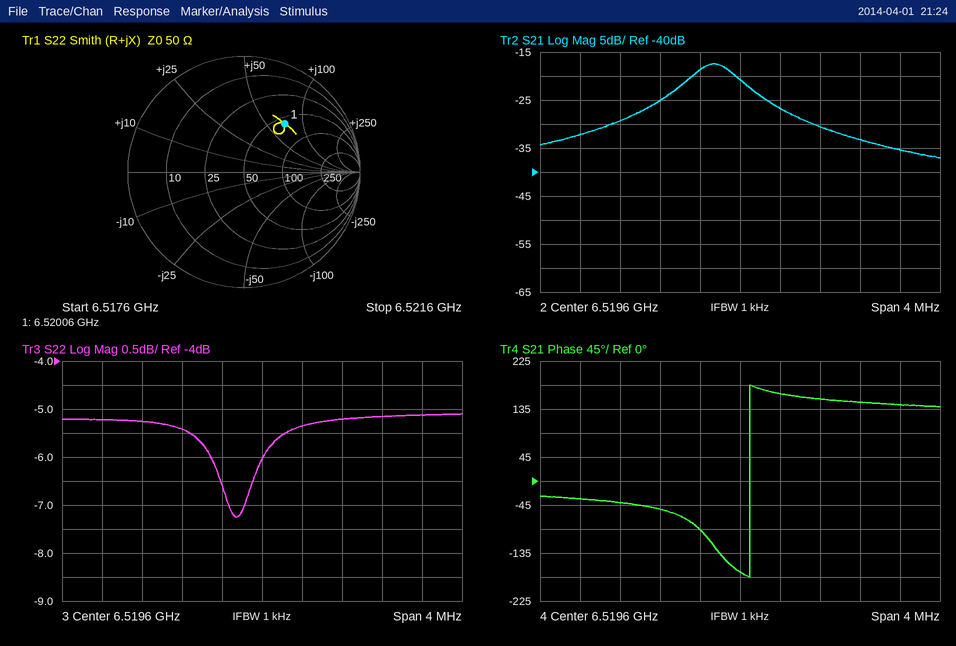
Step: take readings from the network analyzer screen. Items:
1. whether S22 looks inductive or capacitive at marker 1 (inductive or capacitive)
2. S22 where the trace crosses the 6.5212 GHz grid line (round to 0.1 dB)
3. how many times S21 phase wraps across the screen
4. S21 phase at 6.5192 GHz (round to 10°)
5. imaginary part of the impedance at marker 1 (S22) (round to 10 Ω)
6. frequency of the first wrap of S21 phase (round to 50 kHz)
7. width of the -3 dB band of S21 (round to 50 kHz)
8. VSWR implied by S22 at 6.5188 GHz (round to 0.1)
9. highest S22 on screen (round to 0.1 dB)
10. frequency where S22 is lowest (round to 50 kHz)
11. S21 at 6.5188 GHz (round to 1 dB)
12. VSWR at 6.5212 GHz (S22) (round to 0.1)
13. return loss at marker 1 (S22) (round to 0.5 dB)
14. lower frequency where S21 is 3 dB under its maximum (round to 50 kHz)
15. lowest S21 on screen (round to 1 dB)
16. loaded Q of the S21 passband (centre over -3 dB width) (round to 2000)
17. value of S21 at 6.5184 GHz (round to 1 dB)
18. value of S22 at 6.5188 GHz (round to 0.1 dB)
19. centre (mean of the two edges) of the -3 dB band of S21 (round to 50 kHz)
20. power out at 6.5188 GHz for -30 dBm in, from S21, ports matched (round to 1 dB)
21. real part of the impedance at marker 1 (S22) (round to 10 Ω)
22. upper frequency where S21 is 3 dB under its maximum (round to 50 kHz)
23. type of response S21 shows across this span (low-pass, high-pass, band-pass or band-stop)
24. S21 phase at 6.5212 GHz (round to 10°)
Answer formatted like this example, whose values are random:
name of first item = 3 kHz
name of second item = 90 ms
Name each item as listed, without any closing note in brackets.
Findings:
whether S22 looks inductive or capacitive at marker 1 = inductive
S22 where the trace crosses the 6.5212 GHz grid line = -5.1 dB
how many times S21 phase wraps across the screen = 1
S21 phase at 6.5192 GHz = -90°
imaginary part of the impedance at marker 1 (S22) = +70 Ω
frequency of the first wrap of S21 phase = 6.51970 GHz
width of the -3 dB band of S21 = 500 kHz
VSWR implied by S22 at 6.5188 GHz = 3.3
highest S22 on screen = -5.1 dB
frequency where S22 is lowest = 6.51935 GHz
S21 at 6.5188 GHz = -25 dB
VSWR at 6.5212 GHz (S22) = 3.5
return loss at marker 1 (S22) = 5.5 dB
lower frequency where S21 is 3 dB under its maximum = 6.51910 GHz
lowest S21 on screen = -37 dB
loaded Q of the S21 passband (centre over -3 dB width) = 14000
value of S21 at 6.5184 GHz = -29 dB
value of S22 at 6.5188 GHz = -5.4 dB
centre (mean of the two edges) of the -3 dB band of S21 = 6.51935 GHz
power out at 6.5188 GHz for -30 dBm in, from S21, ports matched = -55 dBm
real part of the impedance at marker 1 (S22) = 60 Ω
upper frequency where S21 is 3 dB under its maximum = 6.51960 GHz
type of response S21 shows across this span = band-pass
S21 phase at 6.5212 GHz = 140°
